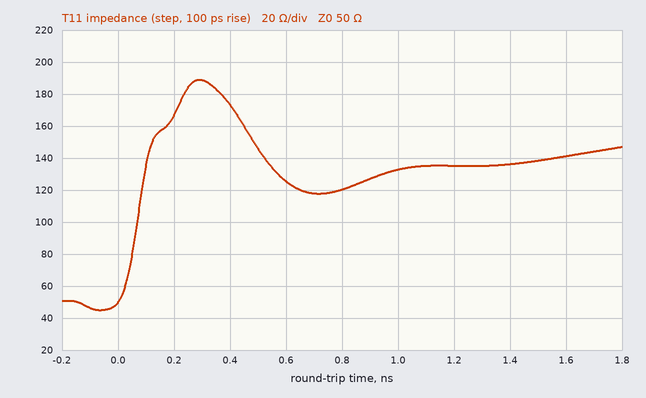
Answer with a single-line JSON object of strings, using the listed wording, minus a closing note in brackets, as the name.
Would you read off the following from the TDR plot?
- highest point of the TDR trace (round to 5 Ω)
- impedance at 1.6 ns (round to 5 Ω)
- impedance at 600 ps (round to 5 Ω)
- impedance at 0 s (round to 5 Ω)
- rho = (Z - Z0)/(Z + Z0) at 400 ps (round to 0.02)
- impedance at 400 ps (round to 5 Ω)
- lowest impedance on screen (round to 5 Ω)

{"highest point of the TDR trace": "190 Ω", "impedance at 1.6 ns": "140 Ω", "impedance at 600 ps": "125 Ω", "impedance at 0 s": "50 Ω", "rho = (Z - Z0)/(Z + Z0) at 400 ps": "+0.56", "impedance at 400 ps": "175 Ω", "lowest impedance on screen": "45 Ω"}
